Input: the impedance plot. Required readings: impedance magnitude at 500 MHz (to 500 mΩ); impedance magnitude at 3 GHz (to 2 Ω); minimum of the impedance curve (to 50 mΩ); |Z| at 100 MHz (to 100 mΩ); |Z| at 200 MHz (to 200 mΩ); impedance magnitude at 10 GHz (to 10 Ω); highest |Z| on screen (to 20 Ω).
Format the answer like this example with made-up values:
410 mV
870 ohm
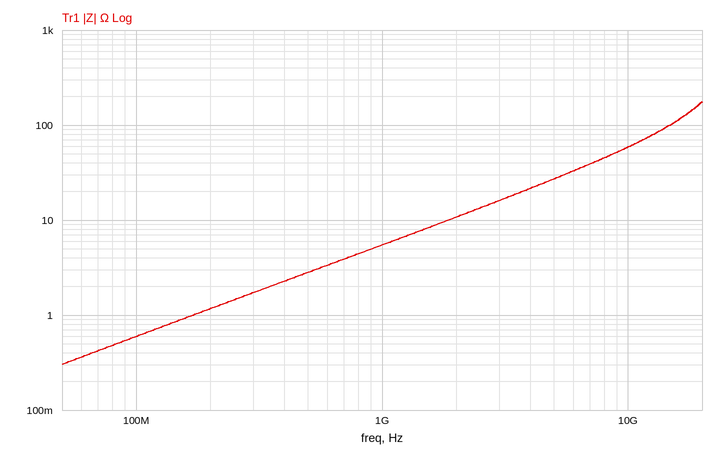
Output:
3.0 Ω
16 Ω
300 mΩ
600 mΩ
1.2 Ω
60 Ω
180 Ω
